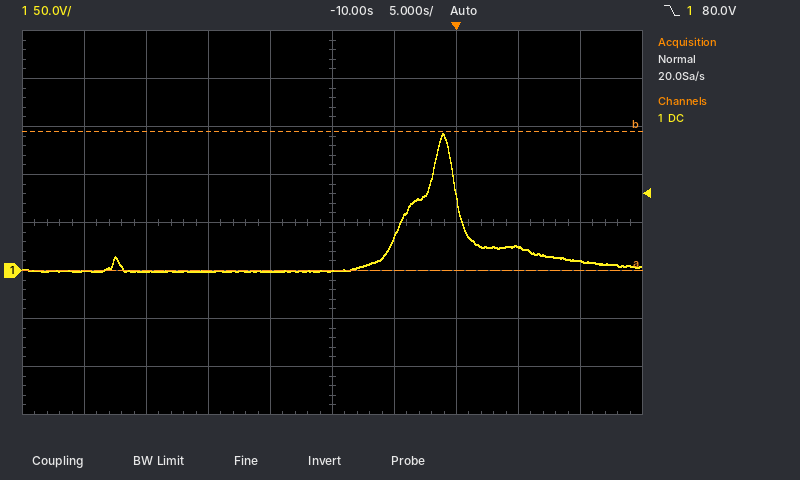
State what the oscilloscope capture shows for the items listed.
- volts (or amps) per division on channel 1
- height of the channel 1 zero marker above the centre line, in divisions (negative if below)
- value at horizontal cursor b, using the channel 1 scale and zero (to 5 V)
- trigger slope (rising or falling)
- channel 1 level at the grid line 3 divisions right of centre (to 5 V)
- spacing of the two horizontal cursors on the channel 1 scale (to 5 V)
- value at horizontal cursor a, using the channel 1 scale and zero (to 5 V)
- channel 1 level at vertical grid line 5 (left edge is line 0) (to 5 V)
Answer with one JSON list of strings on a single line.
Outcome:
["50 V", "-1.0 div", "145 V", "falling", "25 V", "145 V", "0 V", "0 V"]
